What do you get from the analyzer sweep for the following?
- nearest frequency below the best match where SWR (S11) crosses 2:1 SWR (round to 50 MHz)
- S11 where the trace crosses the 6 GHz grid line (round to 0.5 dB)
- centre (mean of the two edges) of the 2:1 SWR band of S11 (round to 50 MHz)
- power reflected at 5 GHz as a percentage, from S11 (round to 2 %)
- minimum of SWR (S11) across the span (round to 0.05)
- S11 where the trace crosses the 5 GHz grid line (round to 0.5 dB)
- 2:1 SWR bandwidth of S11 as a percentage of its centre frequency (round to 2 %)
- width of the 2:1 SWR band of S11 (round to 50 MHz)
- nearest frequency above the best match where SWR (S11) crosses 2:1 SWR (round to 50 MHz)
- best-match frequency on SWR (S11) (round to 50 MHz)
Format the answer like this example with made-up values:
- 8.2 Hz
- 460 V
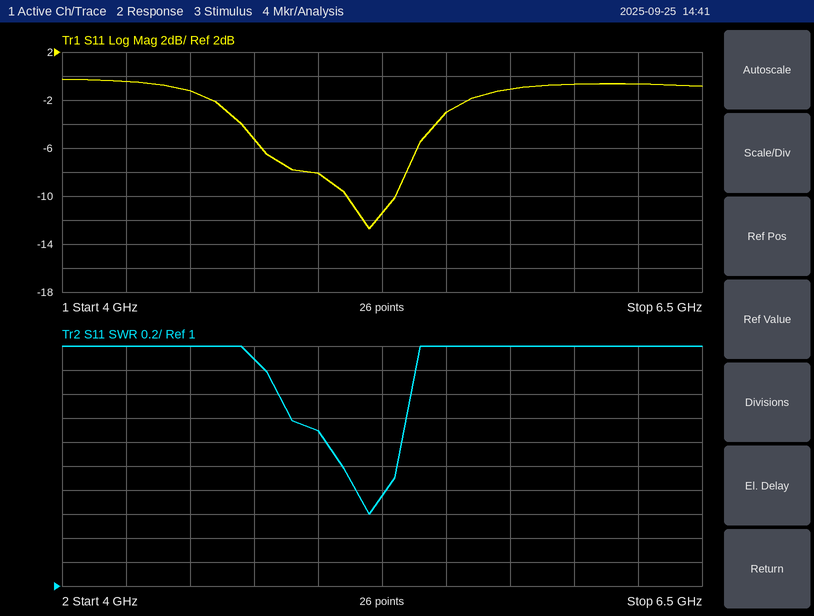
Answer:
- 5.10 GHz
- -0.5 dB
- 5.20 GHz
- 16 %
- 1.60
- -8.0 dB
- 4 %
- 200 MHz
- 5.30 GHz
- 5.20 GHz
